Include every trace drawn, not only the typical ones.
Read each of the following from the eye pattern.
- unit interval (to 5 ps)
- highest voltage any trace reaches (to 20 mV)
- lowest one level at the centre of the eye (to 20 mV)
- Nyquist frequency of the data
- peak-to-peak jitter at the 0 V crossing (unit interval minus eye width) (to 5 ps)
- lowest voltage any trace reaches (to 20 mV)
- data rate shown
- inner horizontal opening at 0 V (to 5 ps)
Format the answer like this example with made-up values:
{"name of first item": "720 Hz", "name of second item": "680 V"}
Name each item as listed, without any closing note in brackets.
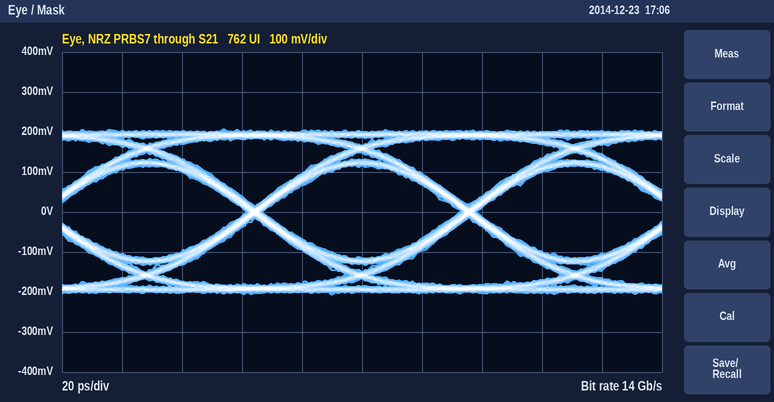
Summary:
{"unit interval": "70 ps", "highest voltage any trace reaches": "200 mV", "lowest one level at the centre of the eye": "120 mV", "Nyquist frequency of the data": "7 GHz", "peak-to-peak jitter at the 0 V crossing (unit interval minus eye width)": "5 ps", "lowest voltage any trace reaches": "-200 mV", "data rate shown": "14 Gb/s", "inner horizontal opening at 0 V": "65 ps"}
